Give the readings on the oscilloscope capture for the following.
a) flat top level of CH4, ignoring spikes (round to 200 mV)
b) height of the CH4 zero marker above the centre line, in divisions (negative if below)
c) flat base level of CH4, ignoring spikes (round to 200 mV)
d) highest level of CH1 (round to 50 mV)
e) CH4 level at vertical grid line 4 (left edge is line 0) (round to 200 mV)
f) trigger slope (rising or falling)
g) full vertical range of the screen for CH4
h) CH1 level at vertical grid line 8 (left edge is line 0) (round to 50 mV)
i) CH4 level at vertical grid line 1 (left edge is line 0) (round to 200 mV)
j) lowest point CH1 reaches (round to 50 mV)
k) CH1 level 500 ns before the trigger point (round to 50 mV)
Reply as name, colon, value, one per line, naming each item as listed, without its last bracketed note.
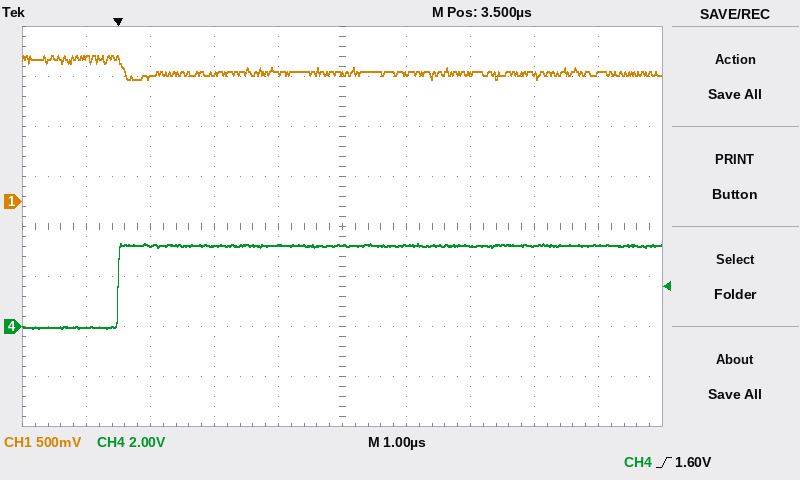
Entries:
flat top level of CH4, ignoring spikes: 3.2 V
height of the CH4 zero marker above the centre line, in divisions: -2.0 div
flat base level of CH4, ignoring spikes: 0.0 V
highest level of CH1: 1.45 V
CH4 level at vertical grid line 4 (left edge is line 0): 3.2 V
trigger slope: rising
full vertical range of the screen for CH4: 16 V
CH1 level at vertical grid line 8 (left edge is line 0): 1.25 V
CH4 level at vertical grid line 1 (left edge is line 0): 0.0 V
lowest point CH1 reaches: 1.20 V
CH1 level 500 ns before the trigger point: 1.45 V
